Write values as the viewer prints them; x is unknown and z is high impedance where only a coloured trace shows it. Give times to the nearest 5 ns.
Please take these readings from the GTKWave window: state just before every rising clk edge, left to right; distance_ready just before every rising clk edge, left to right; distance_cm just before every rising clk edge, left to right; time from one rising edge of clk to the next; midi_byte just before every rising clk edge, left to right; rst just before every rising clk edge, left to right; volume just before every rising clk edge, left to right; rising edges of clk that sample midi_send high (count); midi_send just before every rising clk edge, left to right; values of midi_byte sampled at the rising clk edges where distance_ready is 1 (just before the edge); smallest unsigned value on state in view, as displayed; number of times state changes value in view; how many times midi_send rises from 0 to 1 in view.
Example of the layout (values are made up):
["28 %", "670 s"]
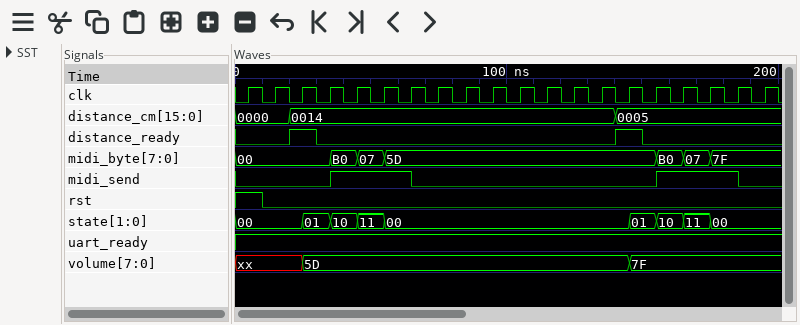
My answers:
["00, 00, 00, 01, 10, 11, 00, 00, 00, 00, 00, 00, 00, 00, 00, 01, 10, 11, 00, 00", "0 0 1 0 0 0 0 0 0 0 0 0 0 0 1 0 0 0 0 0", "0000, 0000, 0014, 0014, 0014, 0014, 0014, 0014, 0014, 0014, 0014, 0014, 0014, 0014, 0005, 0005, 0005, 0005, 0005, 0005", "10 ns", "00, 00, 00, 00, B0, 07, 5D, 5D, 5D, 5D, 5D, 5D, 5D, 5D, 5D, 5D, B0, 07, 7F, 7F", "1 0 0 0 0 0 0 0 0 0 0 0 0 0 0 0 0 0 0 0", "xx, xx, xx, 5D, 5D, 5D, 5D, 5D, 5D, 5D, 5D, 5D, 5D, 5D, 5D, 7F, 7F, 7F, 7F, 7F", "6", "0 0 0 0 1 1 1 0 0 0 0 0 0 0 0 0 1 1 1 0", "00, 5D", "00", "8", "2"]
